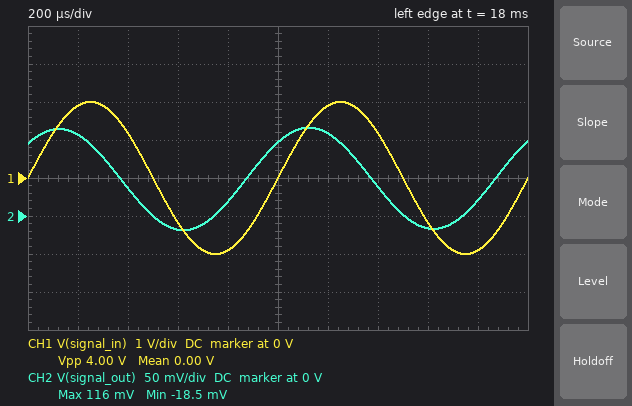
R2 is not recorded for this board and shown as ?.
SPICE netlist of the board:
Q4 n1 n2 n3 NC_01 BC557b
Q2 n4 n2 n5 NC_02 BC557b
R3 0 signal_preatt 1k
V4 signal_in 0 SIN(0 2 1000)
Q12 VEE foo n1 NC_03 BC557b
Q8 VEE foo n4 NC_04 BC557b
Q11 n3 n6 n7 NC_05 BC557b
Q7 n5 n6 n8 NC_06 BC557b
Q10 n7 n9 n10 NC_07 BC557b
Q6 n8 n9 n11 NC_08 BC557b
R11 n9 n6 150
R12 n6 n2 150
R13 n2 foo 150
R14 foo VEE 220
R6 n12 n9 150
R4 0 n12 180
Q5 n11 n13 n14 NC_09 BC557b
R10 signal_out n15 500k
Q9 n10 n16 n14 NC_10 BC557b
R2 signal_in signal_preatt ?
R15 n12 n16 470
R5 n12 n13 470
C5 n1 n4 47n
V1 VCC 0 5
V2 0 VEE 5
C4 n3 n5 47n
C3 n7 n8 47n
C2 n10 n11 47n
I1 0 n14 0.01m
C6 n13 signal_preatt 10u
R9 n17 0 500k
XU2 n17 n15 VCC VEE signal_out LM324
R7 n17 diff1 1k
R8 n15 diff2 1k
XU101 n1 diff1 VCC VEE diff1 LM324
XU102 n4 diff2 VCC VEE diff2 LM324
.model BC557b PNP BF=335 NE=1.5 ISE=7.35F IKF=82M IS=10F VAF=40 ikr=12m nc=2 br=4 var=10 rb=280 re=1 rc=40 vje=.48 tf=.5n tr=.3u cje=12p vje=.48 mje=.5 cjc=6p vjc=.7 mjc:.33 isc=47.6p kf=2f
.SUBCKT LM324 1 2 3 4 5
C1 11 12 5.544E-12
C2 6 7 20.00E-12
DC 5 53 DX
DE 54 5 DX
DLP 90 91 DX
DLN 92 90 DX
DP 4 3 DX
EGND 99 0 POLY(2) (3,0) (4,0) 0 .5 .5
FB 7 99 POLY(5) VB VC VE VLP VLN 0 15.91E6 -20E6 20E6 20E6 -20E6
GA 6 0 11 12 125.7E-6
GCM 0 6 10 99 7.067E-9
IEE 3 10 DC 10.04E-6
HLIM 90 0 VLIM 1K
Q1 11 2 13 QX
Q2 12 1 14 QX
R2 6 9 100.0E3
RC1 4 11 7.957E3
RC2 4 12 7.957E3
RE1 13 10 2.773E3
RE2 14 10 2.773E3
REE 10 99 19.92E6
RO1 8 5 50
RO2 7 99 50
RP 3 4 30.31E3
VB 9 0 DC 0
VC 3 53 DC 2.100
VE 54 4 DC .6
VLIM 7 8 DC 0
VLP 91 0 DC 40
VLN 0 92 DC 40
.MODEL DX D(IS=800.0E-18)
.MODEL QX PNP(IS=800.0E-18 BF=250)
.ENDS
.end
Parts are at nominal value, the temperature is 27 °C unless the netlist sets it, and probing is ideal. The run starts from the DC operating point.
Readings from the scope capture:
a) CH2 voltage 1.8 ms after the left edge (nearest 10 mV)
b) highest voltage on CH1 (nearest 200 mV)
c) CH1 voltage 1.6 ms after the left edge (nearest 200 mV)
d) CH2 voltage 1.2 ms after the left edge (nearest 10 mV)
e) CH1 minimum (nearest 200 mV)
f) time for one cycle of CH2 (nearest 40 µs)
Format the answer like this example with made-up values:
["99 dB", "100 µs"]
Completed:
["20 mV", "2.0 V", "-1.2 V", "110 mV", "-2.0 V", "1.00 ms"]
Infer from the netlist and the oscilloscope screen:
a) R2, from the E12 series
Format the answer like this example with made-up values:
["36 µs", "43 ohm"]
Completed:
["33 kΩ"]
